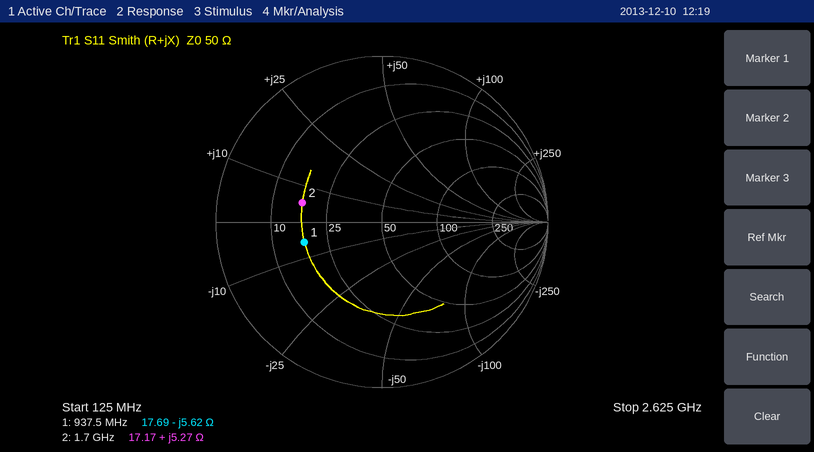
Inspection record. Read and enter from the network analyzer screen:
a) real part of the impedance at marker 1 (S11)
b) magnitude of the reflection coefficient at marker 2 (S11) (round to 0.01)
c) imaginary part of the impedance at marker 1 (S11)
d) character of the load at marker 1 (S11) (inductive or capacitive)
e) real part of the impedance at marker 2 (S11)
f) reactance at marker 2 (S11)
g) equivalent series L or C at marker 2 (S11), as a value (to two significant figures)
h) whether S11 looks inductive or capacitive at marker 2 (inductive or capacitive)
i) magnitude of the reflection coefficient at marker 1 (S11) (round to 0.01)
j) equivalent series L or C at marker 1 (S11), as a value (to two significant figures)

17.69 Ω
0.49
-5.62 Ω
capacitive
17.17 Ω
+5.27 Ω
490 pH
inductive
0.48
30 pF
